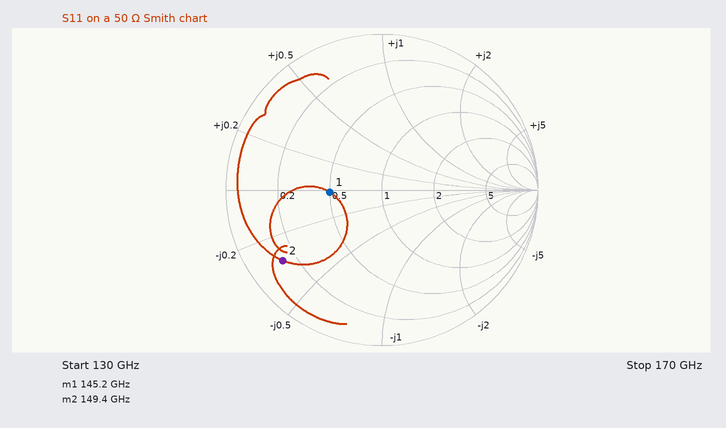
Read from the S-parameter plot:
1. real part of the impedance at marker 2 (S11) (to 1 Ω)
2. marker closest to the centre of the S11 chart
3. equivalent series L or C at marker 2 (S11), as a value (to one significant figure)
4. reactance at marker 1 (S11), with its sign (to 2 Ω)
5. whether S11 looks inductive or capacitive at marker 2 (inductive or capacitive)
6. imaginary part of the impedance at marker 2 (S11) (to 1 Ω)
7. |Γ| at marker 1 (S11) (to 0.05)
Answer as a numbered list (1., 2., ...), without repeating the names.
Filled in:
1. 7 Ω
2. marker 1
3. 70 fF
4. 0 Ω
5. capacitive
6. -16 Ω
7. 0.35
